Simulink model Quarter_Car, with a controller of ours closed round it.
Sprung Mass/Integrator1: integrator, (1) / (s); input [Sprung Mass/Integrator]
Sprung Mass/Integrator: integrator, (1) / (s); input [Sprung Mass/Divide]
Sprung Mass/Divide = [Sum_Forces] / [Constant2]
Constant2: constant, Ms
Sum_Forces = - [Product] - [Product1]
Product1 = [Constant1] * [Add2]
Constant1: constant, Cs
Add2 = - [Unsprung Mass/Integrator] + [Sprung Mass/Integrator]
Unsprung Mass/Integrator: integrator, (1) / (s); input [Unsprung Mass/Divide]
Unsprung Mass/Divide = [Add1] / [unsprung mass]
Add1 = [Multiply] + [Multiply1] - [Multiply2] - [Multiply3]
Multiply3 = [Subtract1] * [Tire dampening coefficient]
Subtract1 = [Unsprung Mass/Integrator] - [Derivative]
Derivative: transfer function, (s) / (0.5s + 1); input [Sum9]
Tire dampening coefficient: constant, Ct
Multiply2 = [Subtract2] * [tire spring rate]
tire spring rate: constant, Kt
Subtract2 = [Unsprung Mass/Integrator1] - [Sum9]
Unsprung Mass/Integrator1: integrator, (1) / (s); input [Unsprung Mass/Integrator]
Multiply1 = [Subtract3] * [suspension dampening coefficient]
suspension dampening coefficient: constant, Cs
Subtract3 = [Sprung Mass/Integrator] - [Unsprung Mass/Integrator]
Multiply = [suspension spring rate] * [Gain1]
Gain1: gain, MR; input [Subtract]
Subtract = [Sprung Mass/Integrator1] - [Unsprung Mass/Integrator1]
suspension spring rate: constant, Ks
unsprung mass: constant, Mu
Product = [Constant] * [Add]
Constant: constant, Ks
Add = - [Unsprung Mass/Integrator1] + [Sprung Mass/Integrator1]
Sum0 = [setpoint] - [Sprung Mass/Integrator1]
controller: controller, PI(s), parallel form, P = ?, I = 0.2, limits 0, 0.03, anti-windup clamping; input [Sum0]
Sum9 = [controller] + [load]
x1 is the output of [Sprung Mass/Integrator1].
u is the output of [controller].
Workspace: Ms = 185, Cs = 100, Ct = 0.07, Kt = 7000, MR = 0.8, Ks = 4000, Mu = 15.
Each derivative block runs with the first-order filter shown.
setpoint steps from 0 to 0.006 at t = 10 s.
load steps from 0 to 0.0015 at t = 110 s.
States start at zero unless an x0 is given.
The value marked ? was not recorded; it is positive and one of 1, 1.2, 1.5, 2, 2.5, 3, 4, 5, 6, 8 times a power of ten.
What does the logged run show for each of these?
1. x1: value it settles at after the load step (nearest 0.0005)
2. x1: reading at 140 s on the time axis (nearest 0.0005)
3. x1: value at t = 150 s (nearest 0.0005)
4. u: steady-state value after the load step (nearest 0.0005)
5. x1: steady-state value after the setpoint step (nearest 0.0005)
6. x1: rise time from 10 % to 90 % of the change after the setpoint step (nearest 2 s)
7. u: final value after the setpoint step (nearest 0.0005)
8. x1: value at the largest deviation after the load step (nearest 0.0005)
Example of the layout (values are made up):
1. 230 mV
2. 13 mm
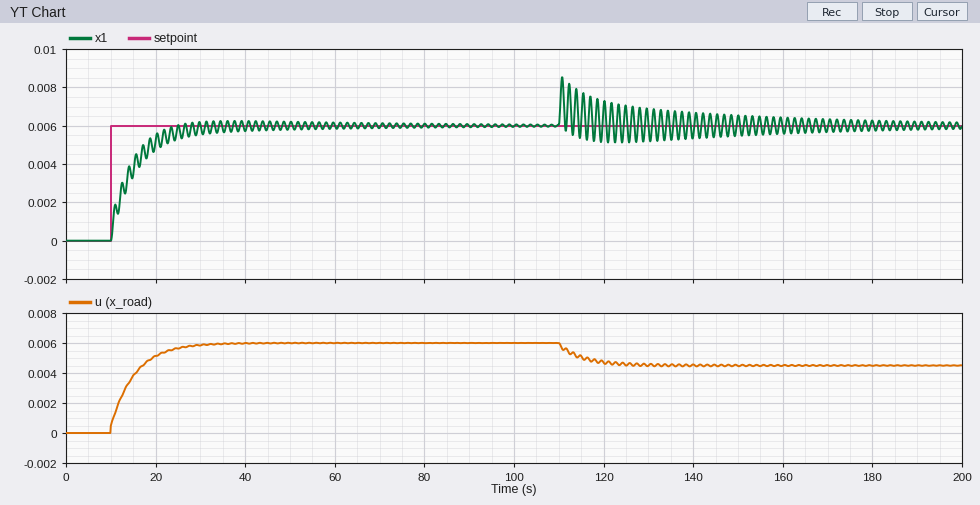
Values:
1. 0.0060
2. 0.0055
3. 0.0065
4. 0.0045
5. 0.0060
6. 10 s
7. 0.0060
8. 0.0085
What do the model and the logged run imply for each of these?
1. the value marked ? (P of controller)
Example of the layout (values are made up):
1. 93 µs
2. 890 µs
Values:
1. 0.08
